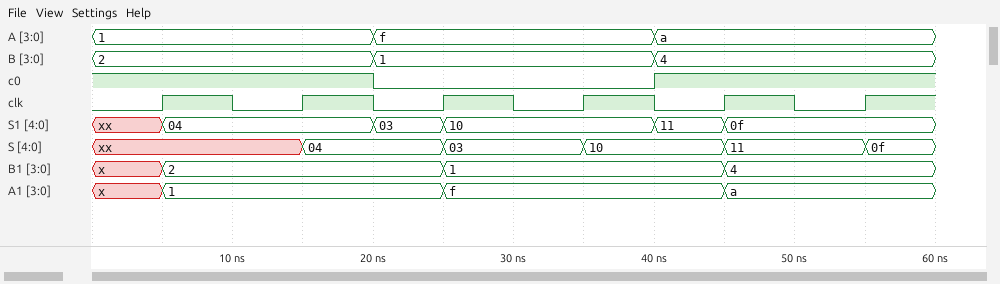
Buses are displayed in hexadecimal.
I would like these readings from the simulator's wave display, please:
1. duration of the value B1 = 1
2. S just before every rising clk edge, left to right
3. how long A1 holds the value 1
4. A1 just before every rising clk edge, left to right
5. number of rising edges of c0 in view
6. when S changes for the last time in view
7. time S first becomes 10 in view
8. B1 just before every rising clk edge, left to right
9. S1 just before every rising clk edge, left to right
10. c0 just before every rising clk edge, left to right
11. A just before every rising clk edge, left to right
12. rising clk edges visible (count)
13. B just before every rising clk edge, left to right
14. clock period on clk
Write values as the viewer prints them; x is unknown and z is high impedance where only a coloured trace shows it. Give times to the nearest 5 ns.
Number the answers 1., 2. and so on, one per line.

1. 20 ns
2. xx, xx, 04, 03, 10, 11
3. 20 ns
4. x, 1, 1, f, f, a
5. 1
6. 55 ns
7. 35 ns
8. x, 2, 2, 1, 1, 4
9. xx, 04, 03, 10, 11, 0f
10. 1 1 0 0 1 1
11. 1, 1, f, f, a, a
12. 6
13. 2, 2, 1, 1, 4, 4
14. 10 ns
